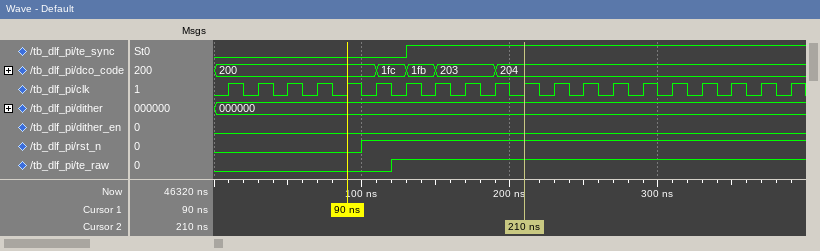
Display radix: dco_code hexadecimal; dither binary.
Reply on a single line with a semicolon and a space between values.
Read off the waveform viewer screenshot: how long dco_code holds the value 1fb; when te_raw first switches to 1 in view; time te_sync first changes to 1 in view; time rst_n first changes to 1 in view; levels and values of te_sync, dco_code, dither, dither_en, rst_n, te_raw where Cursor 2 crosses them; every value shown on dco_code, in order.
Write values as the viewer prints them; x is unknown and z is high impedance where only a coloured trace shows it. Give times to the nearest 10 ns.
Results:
20 ns; 120 ns; 130 ns; 100 ns; te_sync=1, dco_code=204, dither=000000, dither_en=0, rst_n=1, te_raw=1; 200, 1fc, 1fb, 203, 204
